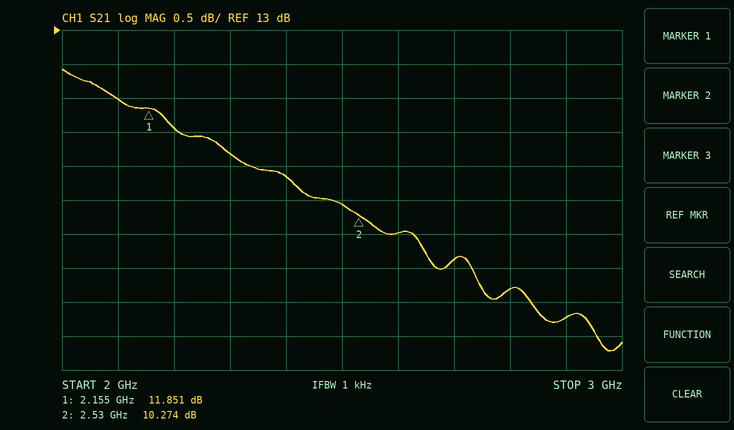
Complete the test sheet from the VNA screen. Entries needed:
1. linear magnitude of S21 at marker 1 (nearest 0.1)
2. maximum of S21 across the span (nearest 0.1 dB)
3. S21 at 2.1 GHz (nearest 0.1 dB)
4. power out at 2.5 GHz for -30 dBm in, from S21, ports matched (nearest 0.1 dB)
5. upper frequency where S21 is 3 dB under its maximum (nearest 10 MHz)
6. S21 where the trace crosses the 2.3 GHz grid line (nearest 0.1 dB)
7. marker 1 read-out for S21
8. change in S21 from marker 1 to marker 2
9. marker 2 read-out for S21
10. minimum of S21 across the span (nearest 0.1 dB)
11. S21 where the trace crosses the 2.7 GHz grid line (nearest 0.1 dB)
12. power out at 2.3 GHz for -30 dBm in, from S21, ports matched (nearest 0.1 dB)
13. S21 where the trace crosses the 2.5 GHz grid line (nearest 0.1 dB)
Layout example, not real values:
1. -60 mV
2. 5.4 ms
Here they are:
1. 3.9
2. 12.4 dB
3. 12.0 dB
4. -19.6 dBm
5. 2.74 GHz
6. 11.2 dB
7. 11.851 dB
8. -1.577 dB
9. 10.274 dB
10. 8.3 dB
11. 9.6 dB
12. -18.8 dBm
13. 10.4 dB
